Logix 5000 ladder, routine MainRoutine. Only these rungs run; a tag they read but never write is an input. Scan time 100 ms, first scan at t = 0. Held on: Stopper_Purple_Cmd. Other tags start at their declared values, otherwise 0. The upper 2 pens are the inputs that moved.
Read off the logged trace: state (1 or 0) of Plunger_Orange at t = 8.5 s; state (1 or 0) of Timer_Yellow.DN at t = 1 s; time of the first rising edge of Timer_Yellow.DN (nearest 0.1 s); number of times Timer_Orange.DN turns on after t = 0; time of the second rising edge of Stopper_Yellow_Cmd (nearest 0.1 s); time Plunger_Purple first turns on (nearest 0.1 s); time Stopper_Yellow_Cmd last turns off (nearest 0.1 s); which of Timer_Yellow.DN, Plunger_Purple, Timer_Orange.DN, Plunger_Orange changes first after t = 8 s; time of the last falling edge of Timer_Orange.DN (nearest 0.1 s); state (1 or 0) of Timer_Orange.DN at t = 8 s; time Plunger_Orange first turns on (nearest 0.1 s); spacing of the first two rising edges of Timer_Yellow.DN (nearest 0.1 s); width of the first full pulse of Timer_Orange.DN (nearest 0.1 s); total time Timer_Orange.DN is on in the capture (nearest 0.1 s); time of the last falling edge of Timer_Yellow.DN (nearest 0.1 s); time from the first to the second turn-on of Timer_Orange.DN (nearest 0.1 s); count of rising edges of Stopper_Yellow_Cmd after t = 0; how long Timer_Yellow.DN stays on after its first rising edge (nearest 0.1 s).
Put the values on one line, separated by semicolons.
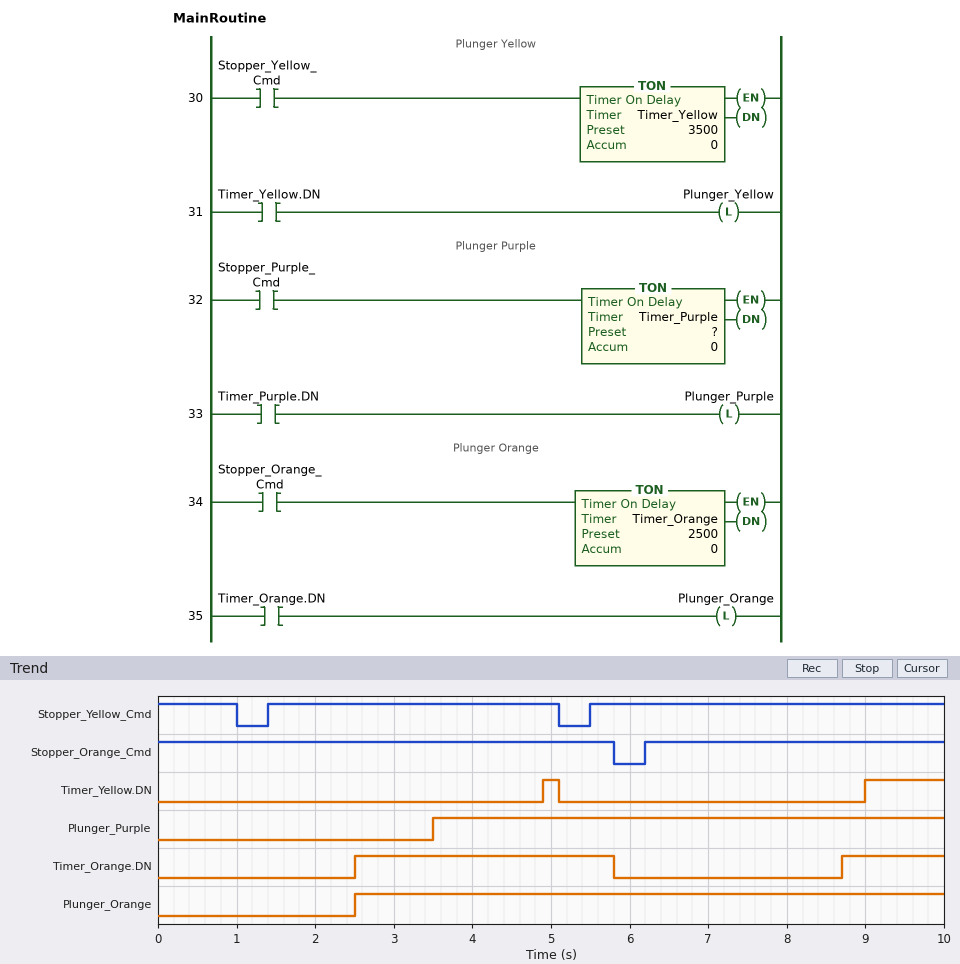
1; 0; 4.9 s; 2; 5.5 s; 3.5 s; 5.1 s; Timer_Orange.DN; 5.8 s; 0; 2.5 s; 4.1 s; 3.3 s; 4.6 s; 5.1 s; 6.2 s; 2; 0.2 s
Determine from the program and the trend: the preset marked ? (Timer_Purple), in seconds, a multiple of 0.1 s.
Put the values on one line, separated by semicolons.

3.5 s
